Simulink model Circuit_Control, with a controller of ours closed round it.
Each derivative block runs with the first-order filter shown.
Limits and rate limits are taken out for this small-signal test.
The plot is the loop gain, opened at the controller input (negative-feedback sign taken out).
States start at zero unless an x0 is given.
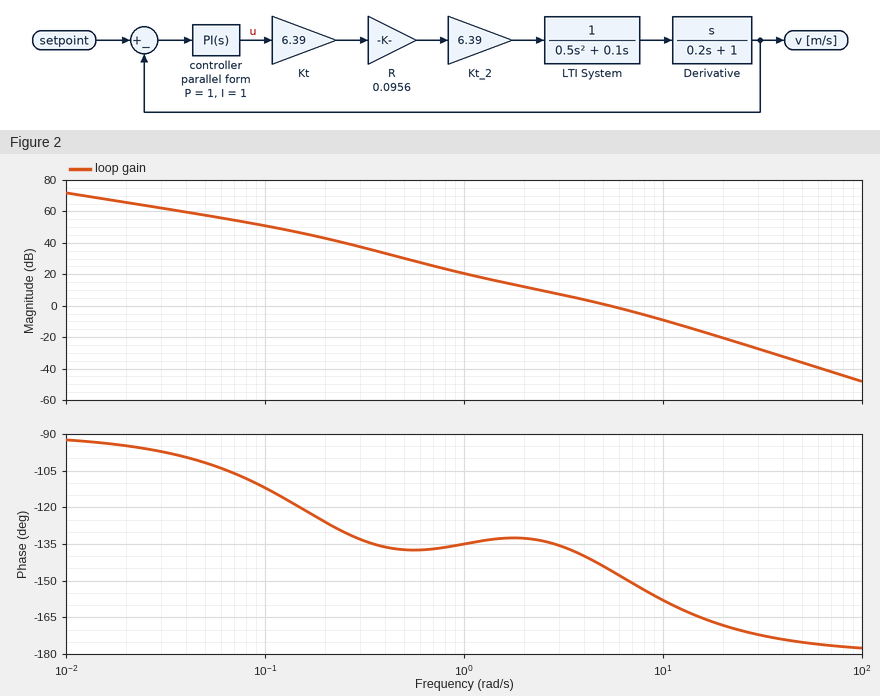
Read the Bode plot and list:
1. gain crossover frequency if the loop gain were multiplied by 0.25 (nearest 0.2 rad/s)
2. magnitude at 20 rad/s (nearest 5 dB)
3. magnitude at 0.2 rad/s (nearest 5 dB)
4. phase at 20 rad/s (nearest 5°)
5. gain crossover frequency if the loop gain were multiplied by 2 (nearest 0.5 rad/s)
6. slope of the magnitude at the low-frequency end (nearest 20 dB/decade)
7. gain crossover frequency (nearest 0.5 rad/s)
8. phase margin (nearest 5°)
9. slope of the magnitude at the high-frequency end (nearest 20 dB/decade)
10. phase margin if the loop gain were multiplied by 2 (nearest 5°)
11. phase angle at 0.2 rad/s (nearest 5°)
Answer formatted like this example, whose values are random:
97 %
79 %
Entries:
2.0 rad/s
-20 dB
45 dB
-170°
8.0 rad/s
-20 dB/decade
5.5 rad/s
35°
-40 dB/decade
25°
-125°
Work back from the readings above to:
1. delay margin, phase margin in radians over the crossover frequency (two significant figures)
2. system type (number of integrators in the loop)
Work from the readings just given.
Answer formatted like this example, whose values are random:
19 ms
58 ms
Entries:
0.11 s
1
